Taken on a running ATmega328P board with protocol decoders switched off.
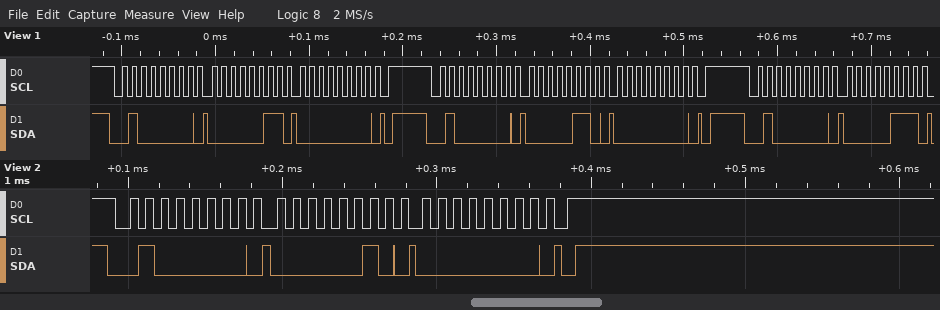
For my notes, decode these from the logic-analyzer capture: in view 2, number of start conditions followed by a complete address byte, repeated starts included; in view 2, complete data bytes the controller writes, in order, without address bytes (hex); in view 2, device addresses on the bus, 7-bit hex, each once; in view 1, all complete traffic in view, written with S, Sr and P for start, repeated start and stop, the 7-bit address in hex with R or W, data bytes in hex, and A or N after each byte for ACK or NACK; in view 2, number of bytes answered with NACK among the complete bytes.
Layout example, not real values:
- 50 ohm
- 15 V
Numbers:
- 1
- 02 00
- 0x20
- S 20W A 03 A 00 A P S 20W A 06 A 00 A P S 20W A 07 A
- 0
